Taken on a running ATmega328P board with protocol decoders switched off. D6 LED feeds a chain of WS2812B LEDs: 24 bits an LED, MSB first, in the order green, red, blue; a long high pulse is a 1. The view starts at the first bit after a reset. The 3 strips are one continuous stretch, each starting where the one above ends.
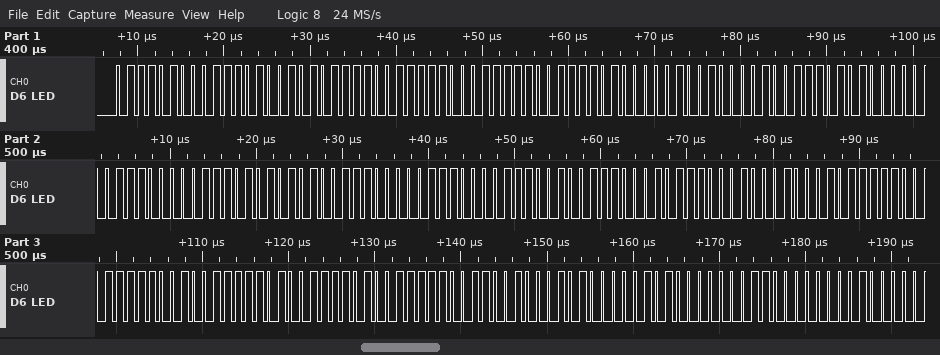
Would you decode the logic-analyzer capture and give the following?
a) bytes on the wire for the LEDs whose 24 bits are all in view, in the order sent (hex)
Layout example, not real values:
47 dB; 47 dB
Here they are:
74 74 AF 3E 3E 7A 09 09 D4 07 07 55 38 38 72 71 71 11 7C 7C 9F 4F 4F 99 14 14 06
